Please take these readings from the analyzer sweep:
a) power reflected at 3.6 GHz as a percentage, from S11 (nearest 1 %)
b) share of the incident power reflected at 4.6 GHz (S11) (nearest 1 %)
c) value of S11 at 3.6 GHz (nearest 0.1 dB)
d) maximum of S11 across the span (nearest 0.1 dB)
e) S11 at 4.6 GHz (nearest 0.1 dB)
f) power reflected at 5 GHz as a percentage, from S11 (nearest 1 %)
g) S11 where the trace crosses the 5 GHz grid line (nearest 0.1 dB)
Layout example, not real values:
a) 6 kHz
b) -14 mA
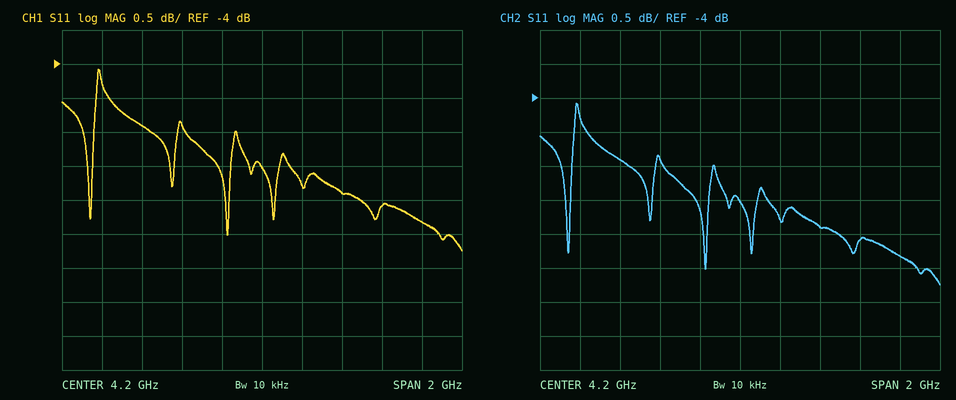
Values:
a) 32 %
b) 26 %
c) -4.9 dB
d) -4.1 dB
e) -5.9 dB
f) 23 %
g) -6.3 dB
